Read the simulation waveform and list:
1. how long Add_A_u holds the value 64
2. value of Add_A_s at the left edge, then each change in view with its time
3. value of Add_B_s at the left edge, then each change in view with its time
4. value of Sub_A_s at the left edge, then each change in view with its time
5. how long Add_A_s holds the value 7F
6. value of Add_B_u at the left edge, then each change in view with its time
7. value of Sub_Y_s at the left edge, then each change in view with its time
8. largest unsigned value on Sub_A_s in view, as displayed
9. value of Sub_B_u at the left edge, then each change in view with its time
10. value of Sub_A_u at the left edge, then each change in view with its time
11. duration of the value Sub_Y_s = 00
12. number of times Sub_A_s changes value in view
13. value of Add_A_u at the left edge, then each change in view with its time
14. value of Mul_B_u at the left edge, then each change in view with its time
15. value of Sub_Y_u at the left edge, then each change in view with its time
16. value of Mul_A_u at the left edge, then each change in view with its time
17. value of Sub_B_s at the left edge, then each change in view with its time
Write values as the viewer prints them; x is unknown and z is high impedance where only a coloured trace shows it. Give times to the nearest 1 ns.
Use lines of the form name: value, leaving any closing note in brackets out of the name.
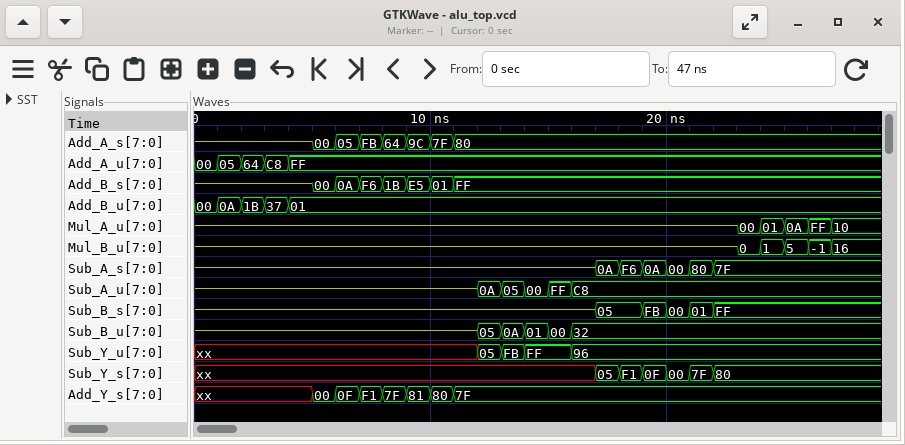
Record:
how long Add_A_u holds the value 64: 1 ns
value of Add_A_s at the left edge, then each change in view with its time: z, 00 at 5 ns, 05 at 6 ns, FB at 7 ns, 64 at 8 ns, 9C at 9 ns, 7F at 10 ns, 80 at 11 ns
value of Add_B_s at the left edge, then each change in view with its time: z, 00 at 5 ns, 0A at 6 ns, F6 at 7 ns, 1B at 8 ns, E5 at 9 ns, 01 at 10 ns, FF at 11 ns
value of Sub_A_s at the left edge, then each change in view with its time: z, 0A at 17 ns, F6 at 18 ns, 0A at 19 ns, 00 at 20 ns, 80 at 21 ns, 7F at 22 ns
how long Add_A_s holds the value 7F: 1 ns
value of Add_B_u at the left edge, then each change in view with its time: 00, 0A at 1 ns, 1B at 2 ns, 37 at 3 ns, 01 at 4 ns
value of Sub_Y_s at the left edge, then each change in view with its time: xx, 05 at 17 ns, F1 at 18 ns, 0F at 19 ns, 00 at 20 ns, 7F at 21 ns, 80 at 22 ns
largest unsigned value on Sub_A_s in view, as displayed: F6
value of Sub_B_u at the left edge, then each change in view with its time: z, 05 at 12 ns, 0A at 13 ns, 01 at 14 ns, 00 at 15 ns, 32 at 16 ns
value of Sub_A_u at the left edge, then each change in view with its time: z, 0A at 12 ns, 05 at 13 ns, 00 at 14 ns, FF at 15 ns, C8 at 16 ns
duration of the value Sub_Y_s = 00: 1 ns
number of times Sub_A_s changes value in view: 6
value of Add_A_u at the left edge, then each change in view with its time: 00, 05 at 1 ns, 64 at 2 ns, C8 at 3 ns, FF at 4 ns
value of Mul_B_u at the left edge, then each change in view with its time: z, 0 at 23 ns, 1 at 24 ns, 5 at 25 ns, -1 at 26 ns, 16 at 27 ns
value of Sub_Y_u at the left edge, then each change in view with its time: xx, 05 at 12 ns, FB at 13 ns, FF at 14 ns, 96 at 16 ns
value of Mul_A_u at the left edge, then each change in view with its time: z, 00 at 23 ns, 01 at 24 ns, 0A at 25 ns, FF at 26 ns, 10 at 27 ns
value of Sub_B_s at the left edge, then each change in view with its time: z, 05 at 17 ns, FB at 19 ns, 00 at 20 ns, 01 at 21 ns, FF at 22 ns
